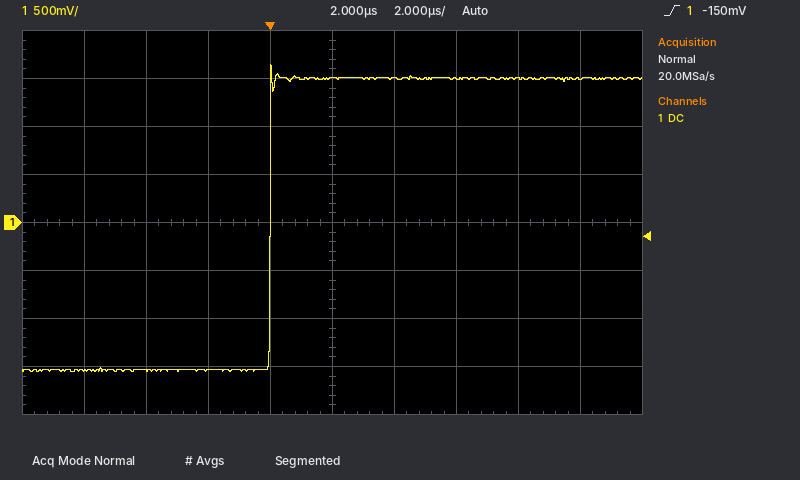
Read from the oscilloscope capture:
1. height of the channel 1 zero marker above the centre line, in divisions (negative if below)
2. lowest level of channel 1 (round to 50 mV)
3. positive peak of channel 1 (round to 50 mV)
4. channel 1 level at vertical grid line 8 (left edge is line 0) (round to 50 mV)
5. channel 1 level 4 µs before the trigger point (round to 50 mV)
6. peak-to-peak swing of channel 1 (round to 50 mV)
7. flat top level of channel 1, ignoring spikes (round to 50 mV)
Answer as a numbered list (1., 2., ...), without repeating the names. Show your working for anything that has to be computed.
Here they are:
1. 0.0 div
2. -1.55 V
3. 1.65 V
4. 1.50 V
5. -1.55 V
6. 1.65 V − (-1.55 V) = 3.20 V
7. 1.50 V
